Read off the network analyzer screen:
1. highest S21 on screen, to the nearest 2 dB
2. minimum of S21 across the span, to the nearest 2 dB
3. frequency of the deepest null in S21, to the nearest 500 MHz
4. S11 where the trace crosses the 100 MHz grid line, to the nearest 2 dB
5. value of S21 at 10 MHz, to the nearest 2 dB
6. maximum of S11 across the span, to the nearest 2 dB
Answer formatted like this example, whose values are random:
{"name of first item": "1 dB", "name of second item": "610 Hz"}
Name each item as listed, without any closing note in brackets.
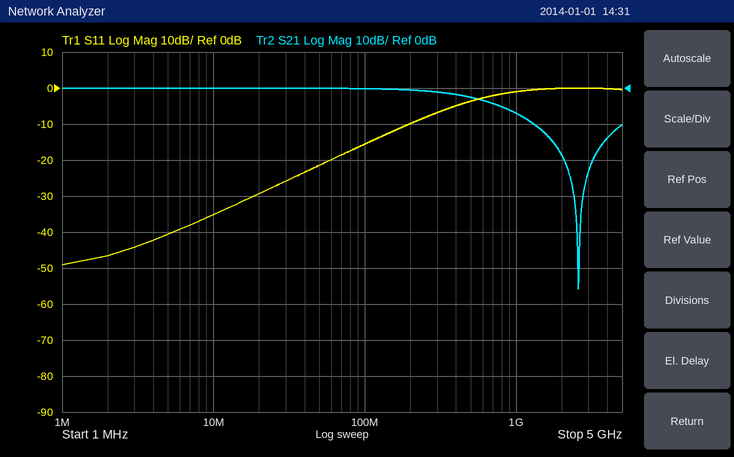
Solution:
{"highest S21 on screen, to the nearest 2 dB": "0 dB", "minimum of S21 across the span, to the nearest 2 dB": "-56 dB", "frequency of the deepest null in S21, to the nearest 500 MHz": "2.5 GHz", "S11 where the trace crosses the 100 MHz grid line, to the nearest 2 dB": "-16 dB", "value of S21 at 10 MHz, to the nearest 2 dB": "0 dB", "maximum of S11 across the span, to the nearest 2 dB": "0 dB"}
